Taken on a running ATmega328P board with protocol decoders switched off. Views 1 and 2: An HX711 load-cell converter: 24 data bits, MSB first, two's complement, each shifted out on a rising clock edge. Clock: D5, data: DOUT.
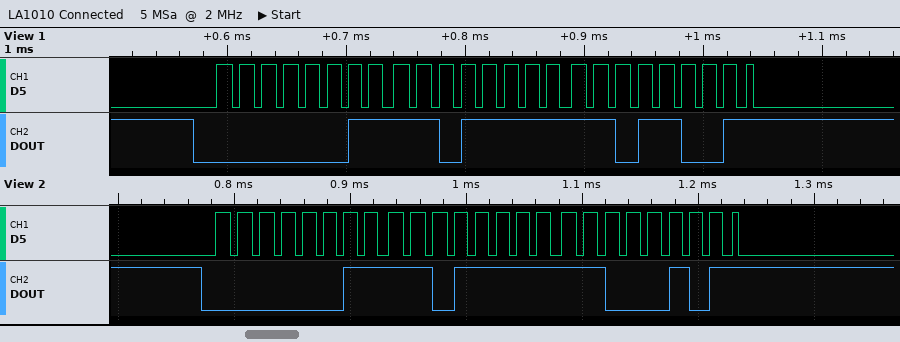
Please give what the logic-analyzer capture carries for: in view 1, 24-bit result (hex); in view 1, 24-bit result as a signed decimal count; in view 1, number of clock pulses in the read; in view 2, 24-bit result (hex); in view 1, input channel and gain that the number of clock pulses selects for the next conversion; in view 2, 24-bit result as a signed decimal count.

0x03DFD9
253913
25
0x03DFC5
channel A, gain 128
253893
